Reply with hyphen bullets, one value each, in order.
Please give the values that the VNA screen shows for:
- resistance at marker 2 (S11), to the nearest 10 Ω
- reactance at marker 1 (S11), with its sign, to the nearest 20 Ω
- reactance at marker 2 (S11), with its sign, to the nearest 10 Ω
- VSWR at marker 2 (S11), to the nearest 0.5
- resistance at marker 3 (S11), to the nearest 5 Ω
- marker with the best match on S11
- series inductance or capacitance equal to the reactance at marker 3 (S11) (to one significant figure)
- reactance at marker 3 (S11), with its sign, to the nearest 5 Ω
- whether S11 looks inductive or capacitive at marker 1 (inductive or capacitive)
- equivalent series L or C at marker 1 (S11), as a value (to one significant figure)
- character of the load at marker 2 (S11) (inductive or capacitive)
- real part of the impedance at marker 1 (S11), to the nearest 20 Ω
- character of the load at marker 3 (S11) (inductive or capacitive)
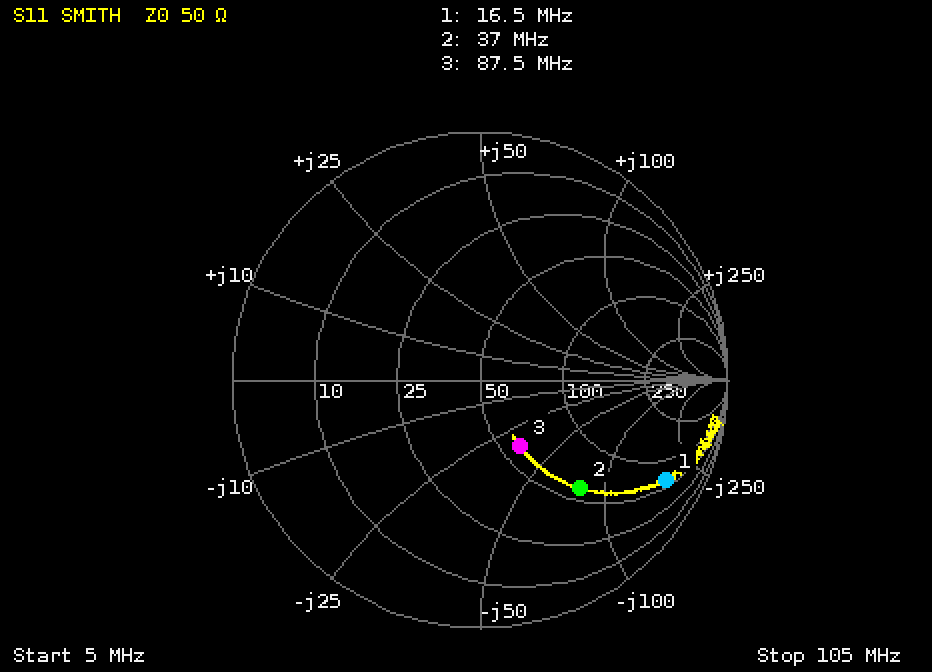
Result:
- 60 Ω
- -180 Ω
- -80 Ω
- 4.0
- 60 Ω
- marker 3
- 50 pF
- -35 Ω
- capacitive
- 50 pF
- capacitive
- 60 Ω
- capacitive
